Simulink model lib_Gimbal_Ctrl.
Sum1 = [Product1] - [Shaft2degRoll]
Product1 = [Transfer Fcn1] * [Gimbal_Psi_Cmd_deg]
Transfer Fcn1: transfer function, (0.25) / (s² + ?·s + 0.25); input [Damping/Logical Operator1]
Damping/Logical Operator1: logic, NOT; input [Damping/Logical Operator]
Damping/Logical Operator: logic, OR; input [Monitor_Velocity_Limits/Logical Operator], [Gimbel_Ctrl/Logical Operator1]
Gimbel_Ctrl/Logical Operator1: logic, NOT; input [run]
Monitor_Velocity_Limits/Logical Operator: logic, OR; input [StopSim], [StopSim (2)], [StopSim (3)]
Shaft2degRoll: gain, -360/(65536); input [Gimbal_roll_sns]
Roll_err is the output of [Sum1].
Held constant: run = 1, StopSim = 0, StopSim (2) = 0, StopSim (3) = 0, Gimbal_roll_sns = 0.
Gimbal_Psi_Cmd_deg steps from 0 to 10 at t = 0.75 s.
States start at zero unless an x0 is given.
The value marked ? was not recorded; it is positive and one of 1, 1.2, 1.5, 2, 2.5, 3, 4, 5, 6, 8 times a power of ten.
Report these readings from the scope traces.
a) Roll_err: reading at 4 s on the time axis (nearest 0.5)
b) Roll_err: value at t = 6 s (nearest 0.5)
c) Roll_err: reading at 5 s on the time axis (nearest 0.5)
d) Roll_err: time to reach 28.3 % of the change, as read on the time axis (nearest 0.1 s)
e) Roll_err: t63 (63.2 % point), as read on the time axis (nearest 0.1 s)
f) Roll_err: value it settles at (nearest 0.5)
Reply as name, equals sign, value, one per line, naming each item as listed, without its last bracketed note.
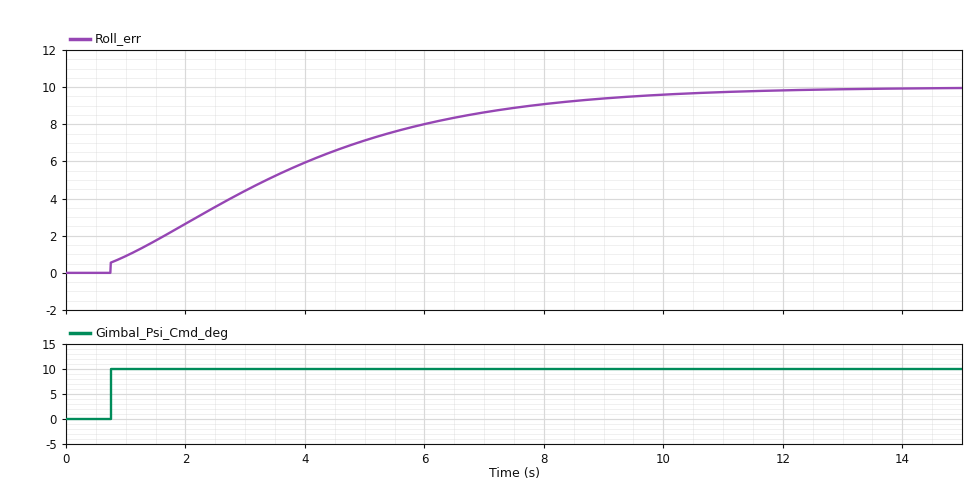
Roll_err: reading at 4 s on the time axis = 6.0
Roll_err: value at t = 6 s = 8.0
Roll_err: reading at 5 s on the time axis = 7.0
Roll_err: time to reach 28.3 % of the change, as read on the time axis = 2.1 s
Roll_err: t63 (63.2 % point), as read on the time axis = 4.3 s
Roll_err: value it settles at = 10.0
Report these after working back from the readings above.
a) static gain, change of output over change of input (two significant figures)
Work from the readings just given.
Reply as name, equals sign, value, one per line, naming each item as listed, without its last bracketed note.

static gain, change of output over change of input = 1.0
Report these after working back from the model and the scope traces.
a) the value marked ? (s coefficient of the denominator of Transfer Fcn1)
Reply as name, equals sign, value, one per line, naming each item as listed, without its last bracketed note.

the value marked ? = 1
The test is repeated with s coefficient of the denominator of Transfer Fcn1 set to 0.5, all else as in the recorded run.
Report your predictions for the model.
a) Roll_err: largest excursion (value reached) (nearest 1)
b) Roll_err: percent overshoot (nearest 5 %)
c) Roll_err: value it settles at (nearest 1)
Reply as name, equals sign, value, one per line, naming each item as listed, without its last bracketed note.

Roll_err: largest excursion (value reached) = 12
Roll_err: percent overshoot = 15 %
Roll_err: value it settles at = 10
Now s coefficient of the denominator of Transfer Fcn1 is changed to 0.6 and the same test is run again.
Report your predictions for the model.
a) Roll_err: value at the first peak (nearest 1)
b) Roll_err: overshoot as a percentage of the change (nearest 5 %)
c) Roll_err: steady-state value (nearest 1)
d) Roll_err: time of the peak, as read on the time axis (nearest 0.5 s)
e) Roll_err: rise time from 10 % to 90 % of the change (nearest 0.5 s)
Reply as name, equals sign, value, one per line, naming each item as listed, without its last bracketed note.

Roll_err: value at the first peak = 11
Roll_err: overshoot as a percentage of the change = 10 %
Roll_err: steady-state value = 10
Roll_err: time of the peak, as read on the time axis = 8.0 s
Roll_err: rise time from 10 % to 90 % of the change = 3.5 s
